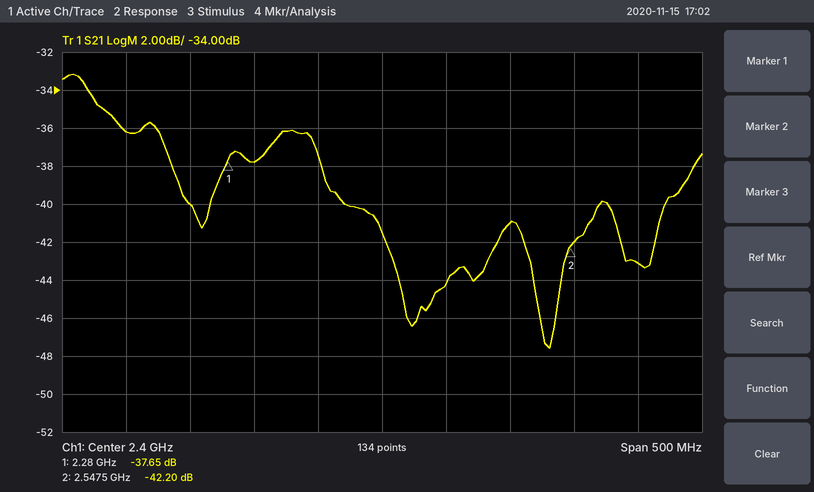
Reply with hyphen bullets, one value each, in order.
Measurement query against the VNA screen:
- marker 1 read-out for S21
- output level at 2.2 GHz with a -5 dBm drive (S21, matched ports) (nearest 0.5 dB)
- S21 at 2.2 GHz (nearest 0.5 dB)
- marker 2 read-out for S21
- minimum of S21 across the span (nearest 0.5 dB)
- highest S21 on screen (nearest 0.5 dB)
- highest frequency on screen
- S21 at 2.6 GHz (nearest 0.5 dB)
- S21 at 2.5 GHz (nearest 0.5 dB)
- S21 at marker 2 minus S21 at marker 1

- -37.65 dB
- -41.0 dBm
- -36.0 dB
- -42.20 dB
- -47.5 dB
- -33.0 dB
- 2.65 GHz
- -43.0 dB
- -41.0 dB
- -4.55 dB
